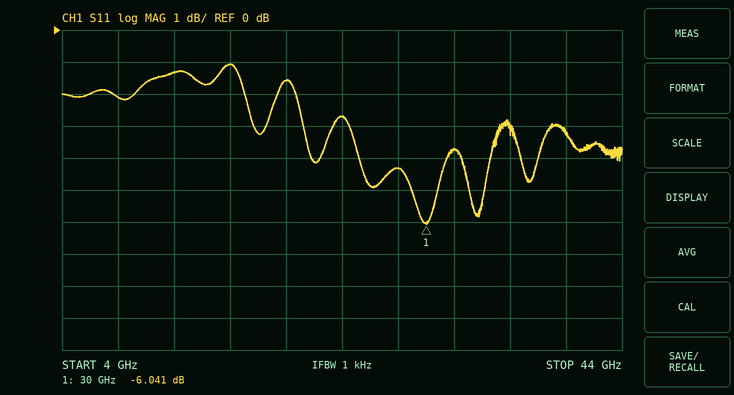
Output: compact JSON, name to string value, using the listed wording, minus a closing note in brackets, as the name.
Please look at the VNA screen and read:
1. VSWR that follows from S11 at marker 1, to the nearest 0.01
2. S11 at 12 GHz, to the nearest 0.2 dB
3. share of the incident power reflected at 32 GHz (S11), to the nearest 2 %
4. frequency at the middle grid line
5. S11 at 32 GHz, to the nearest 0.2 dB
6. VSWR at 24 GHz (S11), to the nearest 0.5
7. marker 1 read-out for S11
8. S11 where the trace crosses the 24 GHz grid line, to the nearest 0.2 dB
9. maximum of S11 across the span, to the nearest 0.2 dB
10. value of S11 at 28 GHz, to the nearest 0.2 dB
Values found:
{"VSWR that follows from S11 at marker 1, to the nearest 0.01": "2.99", "S11 at 12 GHz, to the nearest 0.2 dB": "-1.4 dB", "share of the incident power reflected at 32 GHz (S11), to the nearest 2 %": "42 %", "frequency at the middle grid line": "24 GHz", "S11 at 32 GHz, to the nearest 0.2 dB": "-3.8 dB", "VSWR at 24 GHz (S11), to the nearest 0.5": "6.5", "marker 1 read-out for S11": "-6.041 dB", "S11 where the trace crosses the 24 GHz grid line, to the nearest 0.2 dB": "-2.6 dB", "maximum of S11 across the span, to the nearest 0.2 dB": "-1.0 dB", "value of S11 at 28 GHz, to the nearest 0.2 dB": "-4.4 dB"}
